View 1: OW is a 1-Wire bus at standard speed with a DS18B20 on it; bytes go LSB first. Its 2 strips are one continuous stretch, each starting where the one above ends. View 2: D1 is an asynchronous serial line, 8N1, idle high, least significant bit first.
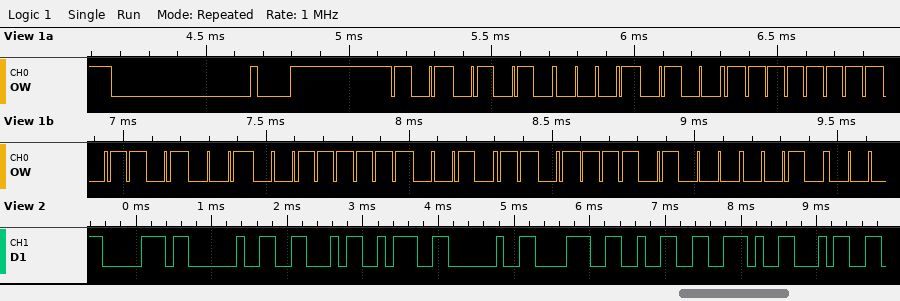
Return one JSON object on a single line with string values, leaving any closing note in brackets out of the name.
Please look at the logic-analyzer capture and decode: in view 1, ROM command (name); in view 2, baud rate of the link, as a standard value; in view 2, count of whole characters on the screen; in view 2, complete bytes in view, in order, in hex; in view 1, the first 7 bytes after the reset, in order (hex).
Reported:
{"in view 1, ROM command": "Match ROM", "in view 2, baud rate of the link, as a standard value": "9600 baud", "in view 2, count of whole characters on the screen": "9", "in view 2, complete bytes in view, in order, in hex": "70 20 46 3A 20 38 32 2E 34", "in view 1, the first 7 bytes after the reset, in order": "55 28 FF 96 FC B4 17"}
